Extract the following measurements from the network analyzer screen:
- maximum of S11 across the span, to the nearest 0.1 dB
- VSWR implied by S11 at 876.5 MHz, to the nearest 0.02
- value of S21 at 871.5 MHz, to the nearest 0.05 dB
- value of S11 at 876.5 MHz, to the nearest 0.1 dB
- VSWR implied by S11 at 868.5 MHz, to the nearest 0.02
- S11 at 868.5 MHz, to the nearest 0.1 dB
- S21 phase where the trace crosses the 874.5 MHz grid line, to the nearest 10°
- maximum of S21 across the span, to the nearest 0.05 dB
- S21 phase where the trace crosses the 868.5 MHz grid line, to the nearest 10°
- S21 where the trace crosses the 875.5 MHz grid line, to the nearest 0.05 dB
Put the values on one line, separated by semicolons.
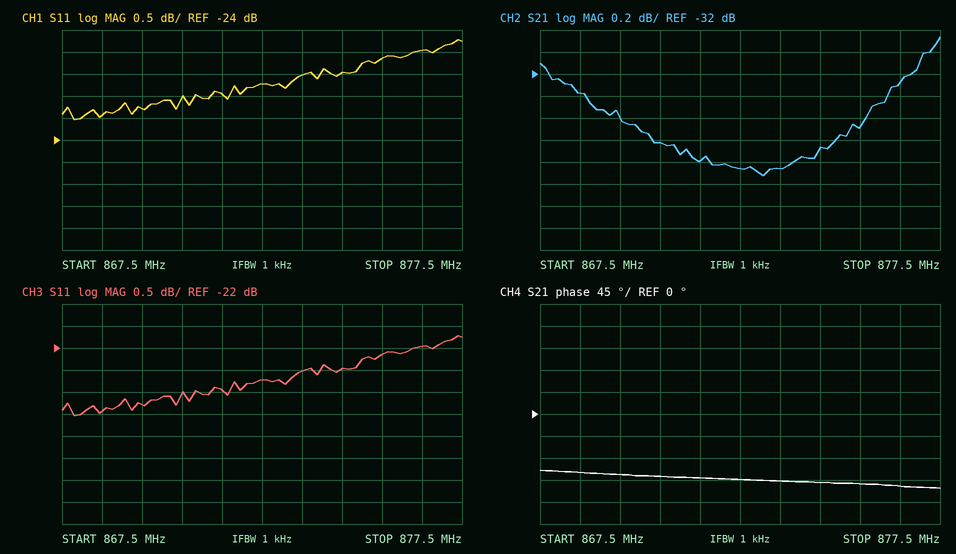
-21.7 dB; 1.18; -32.80 dB; -22.0 dB; 1.14; -23.4 dB; -140°; -31.65 dB; -120°; -32.50 dB
